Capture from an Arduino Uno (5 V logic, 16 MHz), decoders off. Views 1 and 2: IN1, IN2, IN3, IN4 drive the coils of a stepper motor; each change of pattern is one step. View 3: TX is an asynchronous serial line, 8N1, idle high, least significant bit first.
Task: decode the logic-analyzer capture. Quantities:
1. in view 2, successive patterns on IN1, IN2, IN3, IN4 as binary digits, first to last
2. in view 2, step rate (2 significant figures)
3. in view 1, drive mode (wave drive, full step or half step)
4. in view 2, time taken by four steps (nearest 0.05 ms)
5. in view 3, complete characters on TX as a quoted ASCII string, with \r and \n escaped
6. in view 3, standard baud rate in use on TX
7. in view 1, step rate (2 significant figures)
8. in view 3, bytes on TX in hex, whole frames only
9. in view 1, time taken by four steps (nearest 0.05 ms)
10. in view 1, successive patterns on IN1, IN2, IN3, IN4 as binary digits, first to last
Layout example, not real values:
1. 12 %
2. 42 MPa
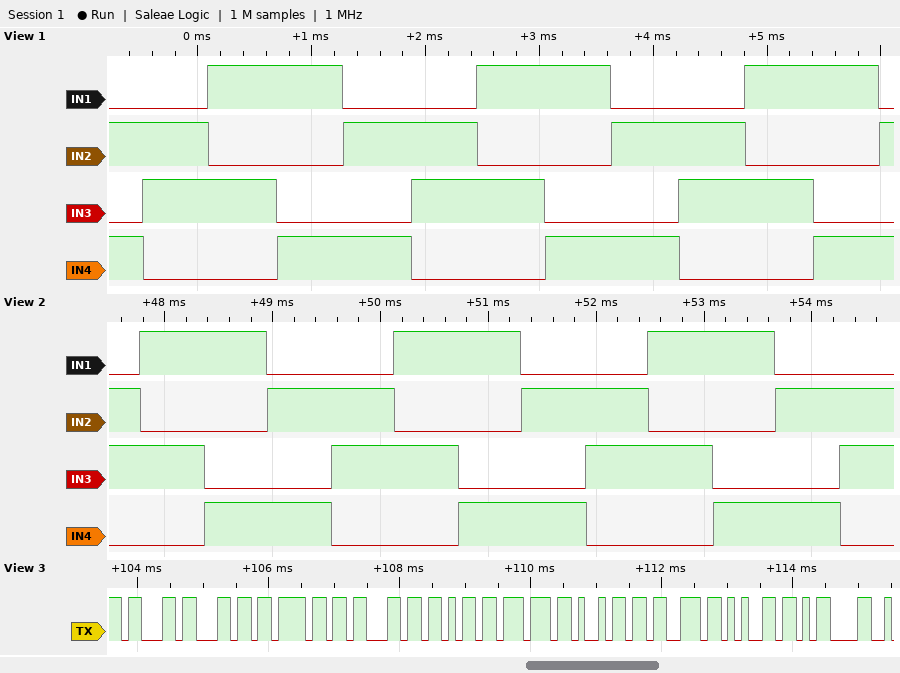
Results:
1. 0110 1010 1001 0101 0110 1010 1001 0101 0110 1010 1001 0101 0110
2. 1700 steps/s
3. full step
4. 2.35 ms
5. "clockwise\r"
6. 9600 baud
7. 1700 steps/s
8. 63 6C 6F 63 6B 77 69 73 65 0D
9. 2.35 ms
10. 0101 0110 1010 1001 0101 0110 1010 1001 0101 0110 1010 1001 0101
